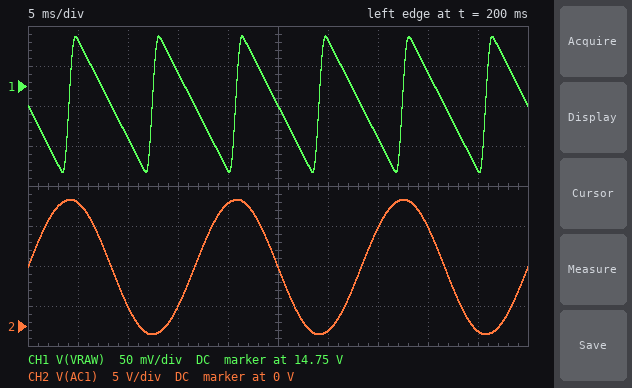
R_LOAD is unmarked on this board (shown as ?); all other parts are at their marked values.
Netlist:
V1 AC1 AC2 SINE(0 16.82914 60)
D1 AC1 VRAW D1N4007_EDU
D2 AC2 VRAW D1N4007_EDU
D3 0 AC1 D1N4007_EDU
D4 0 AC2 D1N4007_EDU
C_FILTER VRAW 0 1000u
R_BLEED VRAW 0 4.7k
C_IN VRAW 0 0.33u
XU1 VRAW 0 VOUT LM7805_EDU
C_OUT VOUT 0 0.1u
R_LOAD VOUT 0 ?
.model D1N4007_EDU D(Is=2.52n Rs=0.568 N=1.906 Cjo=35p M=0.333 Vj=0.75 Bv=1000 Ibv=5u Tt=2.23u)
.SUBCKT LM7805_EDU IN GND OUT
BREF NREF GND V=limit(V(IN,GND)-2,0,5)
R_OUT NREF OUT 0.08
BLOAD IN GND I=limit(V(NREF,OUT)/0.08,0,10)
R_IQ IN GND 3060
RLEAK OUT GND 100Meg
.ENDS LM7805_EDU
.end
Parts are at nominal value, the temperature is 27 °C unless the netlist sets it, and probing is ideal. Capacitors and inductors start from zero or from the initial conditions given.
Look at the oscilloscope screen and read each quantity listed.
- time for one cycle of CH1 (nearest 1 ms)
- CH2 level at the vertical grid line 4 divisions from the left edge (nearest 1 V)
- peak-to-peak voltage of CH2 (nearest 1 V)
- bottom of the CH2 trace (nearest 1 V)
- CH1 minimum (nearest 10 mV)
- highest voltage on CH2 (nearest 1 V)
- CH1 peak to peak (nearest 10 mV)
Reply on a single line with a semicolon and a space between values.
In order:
8 ms; 15 V; 17 V; -1 V; 14.64 V; 16 V; 170 mV
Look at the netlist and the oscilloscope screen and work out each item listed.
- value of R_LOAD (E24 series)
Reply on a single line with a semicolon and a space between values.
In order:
300 Ω
